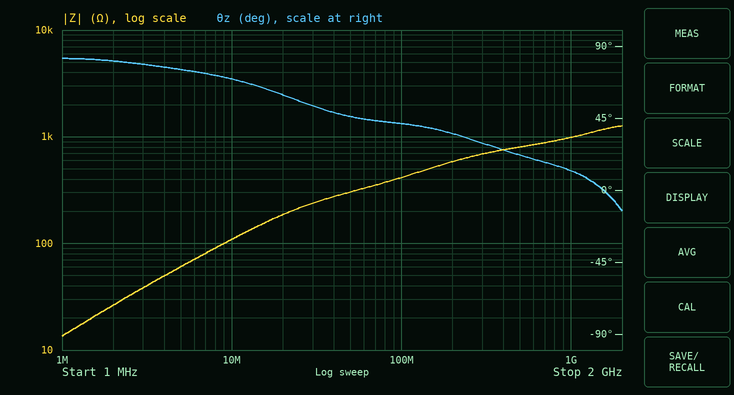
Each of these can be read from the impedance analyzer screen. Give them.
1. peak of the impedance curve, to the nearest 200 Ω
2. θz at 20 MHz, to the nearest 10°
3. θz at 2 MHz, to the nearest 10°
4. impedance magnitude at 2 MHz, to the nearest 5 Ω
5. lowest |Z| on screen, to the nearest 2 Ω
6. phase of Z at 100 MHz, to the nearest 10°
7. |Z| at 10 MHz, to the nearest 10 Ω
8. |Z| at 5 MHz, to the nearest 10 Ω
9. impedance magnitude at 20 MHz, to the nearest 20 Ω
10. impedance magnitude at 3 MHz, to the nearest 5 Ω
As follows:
1.2 kΩ
60°
80°
25 Ω
14 Ω
40°
110 Ω
60 Ω
180 Ω
40 Ω
